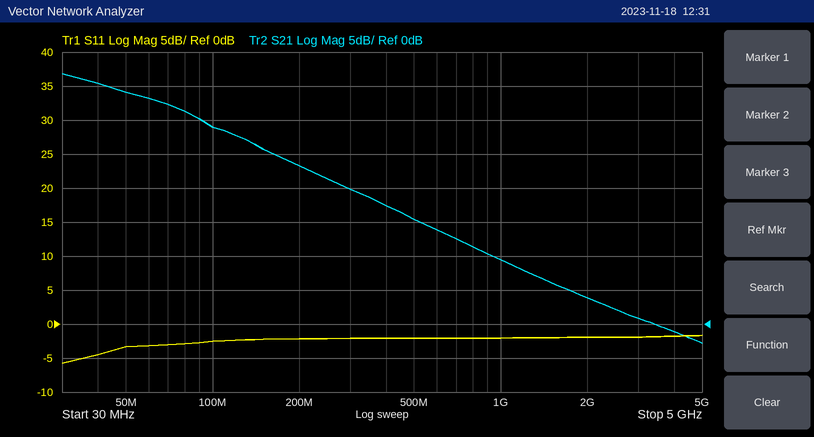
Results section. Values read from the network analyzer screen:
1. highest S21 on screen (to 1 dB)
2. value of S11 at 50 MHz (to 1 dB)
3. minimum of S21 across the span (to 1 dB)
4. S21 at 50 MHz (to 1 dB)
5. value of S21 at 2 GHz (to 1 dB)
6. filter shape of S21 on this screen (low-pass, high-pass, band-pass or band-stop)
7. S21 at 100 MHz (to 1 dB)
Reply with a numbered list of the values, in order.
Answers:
1. 37 dB
2. -3 dB
3. -3 dB
4. 34 dB
5. 4 dB
6. low-pass
7. 29 dB
